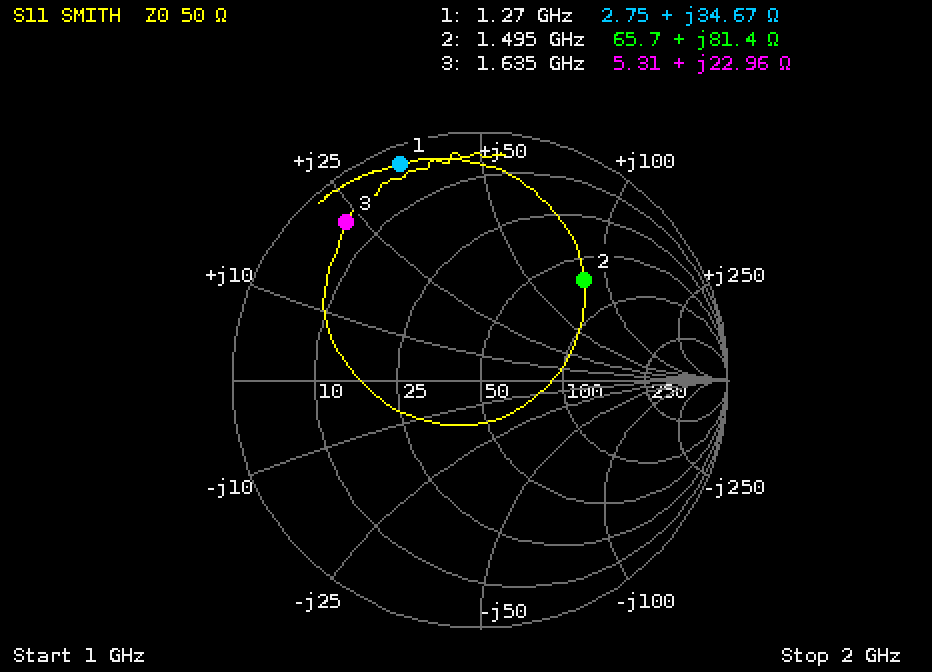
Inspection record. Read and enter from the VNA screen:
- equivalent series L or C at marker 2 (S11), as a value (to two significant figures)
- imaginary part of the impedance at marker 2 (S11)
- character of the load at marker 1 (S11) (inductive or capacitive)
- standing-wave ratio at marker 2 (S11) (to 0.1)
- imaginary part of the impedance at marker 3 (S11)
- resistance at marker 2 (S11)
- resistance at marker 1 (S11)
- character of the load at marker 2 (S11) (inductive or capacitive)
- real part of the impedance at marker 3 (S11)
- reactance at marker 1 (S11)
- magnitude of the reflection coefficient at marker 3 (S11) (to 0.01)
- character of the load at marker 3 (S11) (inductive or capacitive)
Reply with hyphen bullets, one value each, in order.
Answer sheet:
- 8.7 nH
- +81.4 Ω
- inductive
- 3.8
- +22.96 Ω
- 65.7 Ω
- 2.75 Ω
- inductive
- 5.31 Ω
- +34.67 Ω
- 0.84
- inductive
